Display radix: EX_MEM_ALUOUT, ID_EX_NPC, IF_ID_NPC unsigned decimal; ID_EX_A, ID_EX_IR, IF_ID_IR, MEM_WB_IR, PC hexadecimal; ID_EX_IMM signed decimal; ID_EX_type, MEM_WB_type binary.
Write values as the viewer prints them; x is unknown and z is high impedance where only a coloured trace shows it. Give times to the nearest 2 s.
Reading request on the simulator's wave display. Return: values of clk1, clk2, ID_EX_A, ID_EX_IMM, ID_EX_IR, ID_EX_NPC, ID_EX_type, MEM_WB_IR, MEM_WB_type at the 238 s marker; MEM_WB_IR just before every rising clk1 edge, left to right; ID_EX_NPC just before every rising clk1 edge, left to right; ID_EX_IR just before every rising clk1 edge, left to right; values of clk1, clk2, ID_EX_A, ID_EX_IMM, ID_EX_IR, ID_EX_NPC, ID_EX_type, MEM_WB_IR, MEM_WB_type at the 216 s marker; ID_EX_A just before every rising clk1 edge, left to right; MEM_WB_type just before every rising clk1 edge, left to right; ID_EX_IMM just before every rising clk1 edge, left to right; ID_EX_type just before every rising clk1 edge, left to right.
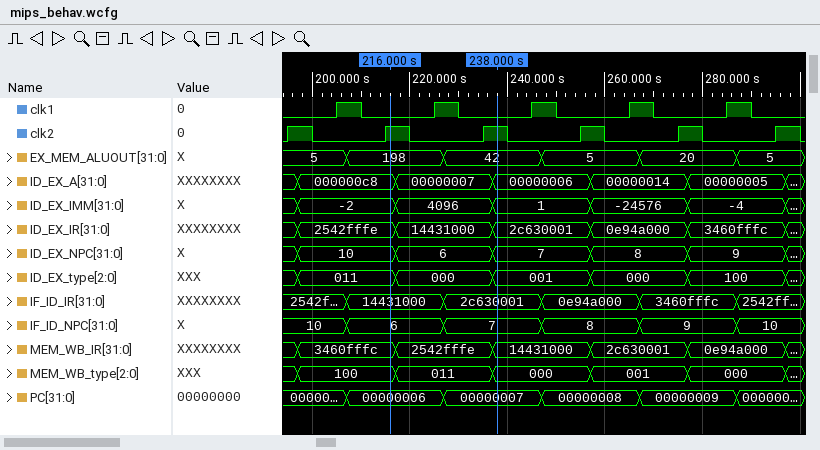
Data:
clk1=0, clk2=1, ID_EX_A=00000006, ID_EX_IMM=1, ID_EX_IR=2c630001, ID_EX_NPC=7, ID_EX_type=001, MEM_WB_IR=14431000, MEM_WB_type=000
3460fffc, 2542fffe, 14431000, 2c630001, 0e94a000
10, 6, 7, 8, 9
2542fffe, 14431000, 2c630001, 0e94a000, 3460fffc
clk1=0, clk2=1, ID_EX_A=000000c8, ID_EX_IMM=-2, ID_EX_IR=2542fffe, ID_EX_NPC=10, ID_EX_type=011, MEM_WB_IR=3460fffc, MEM_WB_type=100
000000c8, 00000007, 00000006, 00000014, 00000005
100, 011, 000, 001, 000
-2, 4096, 1, -24576, -4
011, 000, 001, 000, 100
